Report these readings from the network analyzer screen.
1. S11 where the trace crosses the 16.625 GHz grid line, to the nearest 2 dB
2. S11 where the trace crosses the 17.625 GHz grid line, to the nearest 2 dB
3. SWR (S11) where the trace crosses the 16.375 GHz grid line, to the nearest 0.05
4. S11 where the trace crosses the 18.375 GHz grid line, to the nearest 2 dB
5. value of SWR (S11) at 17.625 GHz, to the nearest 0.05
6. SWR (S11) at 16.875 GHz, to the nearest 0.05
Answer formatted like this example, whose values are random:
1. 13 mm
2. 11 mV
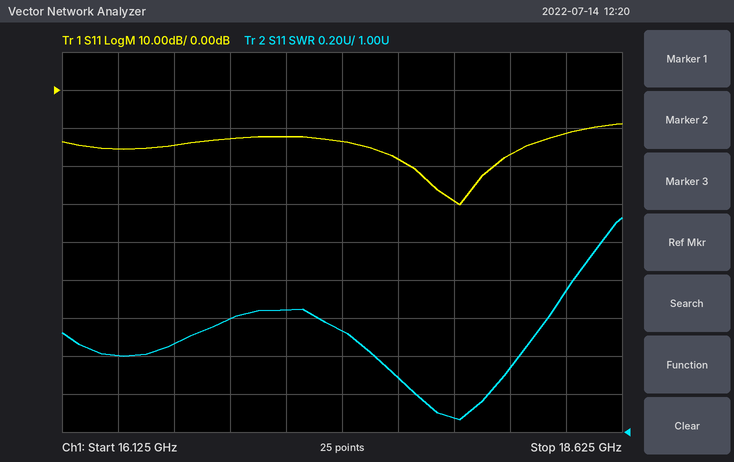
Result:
1. -14 dB
2. -18 dB
3. 1.40
4. -12 dB
5. 1.30
6. 1.60
